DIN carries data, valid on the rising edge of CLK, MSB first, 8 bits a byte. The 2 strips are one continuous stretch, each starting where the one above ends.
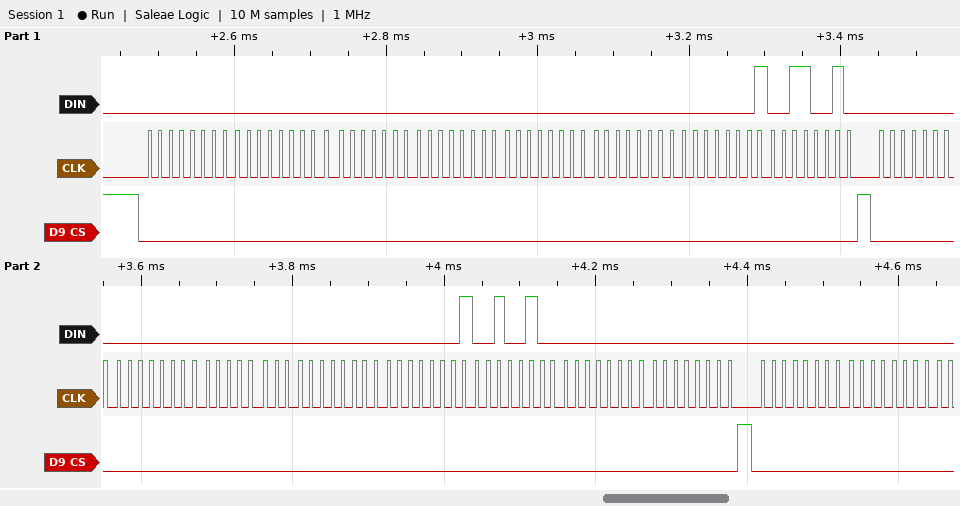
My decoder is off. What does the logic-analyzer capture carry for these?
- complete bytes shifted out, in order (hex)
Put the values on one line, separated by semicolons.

0x00 0x00 0x00 0x00 0x00 0x00 0x01 0x32 0x00 0x00 0x00 0x00 0x01 0x24 0x00 0x00 0x00 0x00
